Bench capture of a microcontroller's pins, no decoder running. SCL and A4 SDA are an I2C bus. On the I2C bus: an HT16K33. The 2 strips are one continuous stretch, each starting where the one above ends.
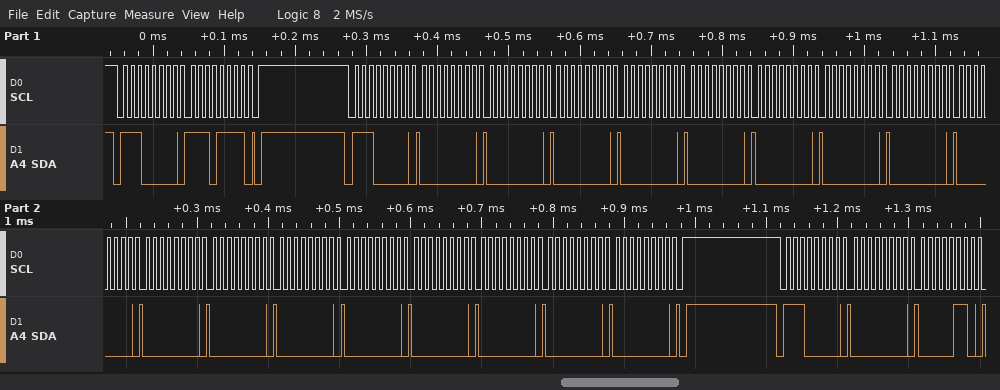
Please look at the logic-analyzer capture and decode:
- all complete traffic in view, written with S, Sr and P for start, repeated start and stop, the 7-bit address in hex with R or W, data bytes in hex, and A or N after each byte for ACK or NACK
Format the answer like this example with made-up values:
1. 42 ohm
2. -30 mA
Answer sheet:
1. S 70W A EF A P S 70W A 00 A 00 A 00 A 00 A 00 A 00 A 00 A 00 A 00 A 00 A 00 A 00 A 00 A 00 A 00 A 00 A 00 A P S 70W A 00 A 06 A
